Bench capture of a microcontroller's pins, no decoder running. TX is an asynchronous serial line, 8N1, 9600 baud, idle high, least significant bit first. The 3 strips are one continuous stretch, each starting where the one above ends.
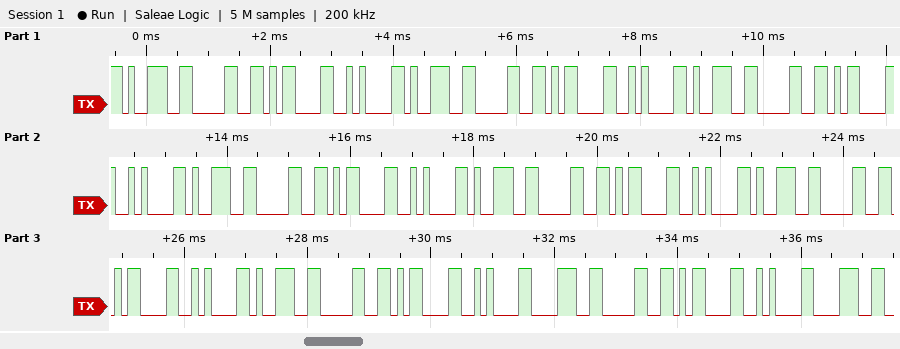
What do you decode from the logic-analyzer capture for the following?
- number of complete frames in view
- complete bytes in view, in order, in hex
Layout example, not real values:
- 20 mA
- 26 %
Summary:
- 33
- 39 30 0D 0A 39 30 0D 0A 39 30 0D 0A 39 30 0D 0A 39 30 0D 0A 39 30 0D 0A 39 30 0D 0A 38 30 0D 0A 38
